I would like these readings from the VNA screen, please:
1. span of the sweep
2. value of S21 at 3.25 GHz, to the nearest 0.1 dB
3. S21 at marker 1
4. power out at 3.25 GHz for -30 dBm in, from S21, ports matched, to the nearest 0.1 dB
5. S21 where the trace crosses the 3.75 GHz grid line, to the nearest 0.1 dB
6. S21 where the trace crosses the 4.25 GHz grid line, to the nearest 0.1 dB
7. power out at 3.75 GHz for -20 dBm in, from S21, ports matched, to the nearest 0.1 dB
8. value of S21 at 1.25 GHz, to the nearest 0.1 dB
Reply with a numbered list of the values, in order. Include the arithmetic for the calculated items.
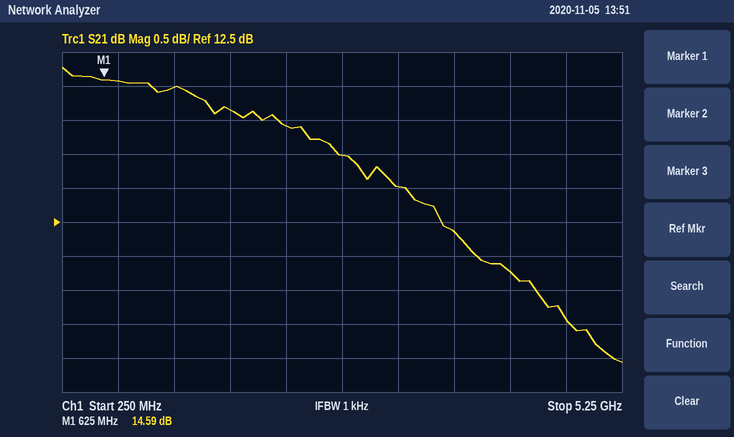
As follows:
1. 5 GHz
2. 13.0 dB
3. 14.59 dB
4. -30 dBm + (13.0 dB) = -17.0 dBm
5. 12.4 dB
6. 11.8 dB
7. -20 dBm + (12.4 dB) = -7.6 dBm
8. 14.5 dB
